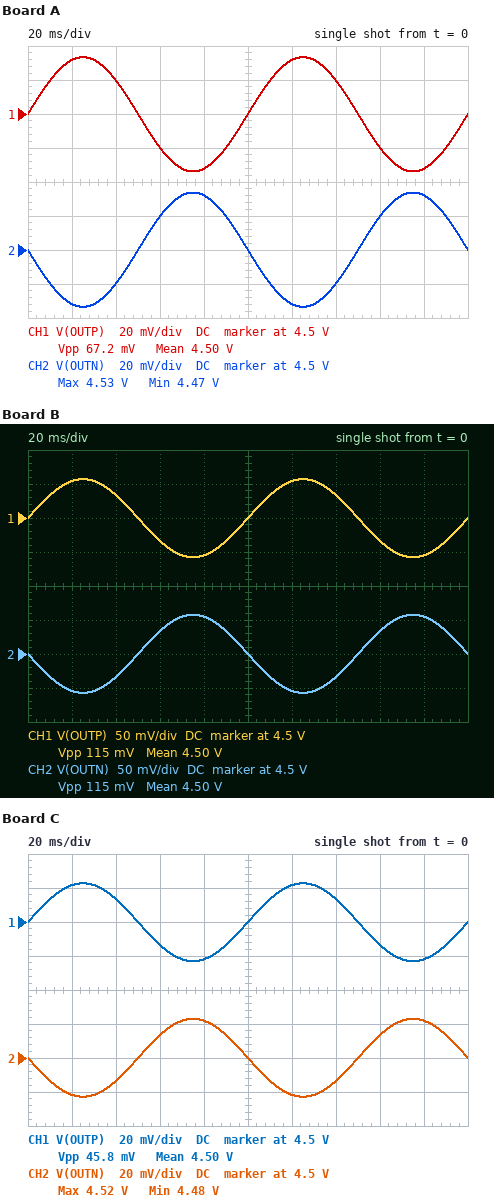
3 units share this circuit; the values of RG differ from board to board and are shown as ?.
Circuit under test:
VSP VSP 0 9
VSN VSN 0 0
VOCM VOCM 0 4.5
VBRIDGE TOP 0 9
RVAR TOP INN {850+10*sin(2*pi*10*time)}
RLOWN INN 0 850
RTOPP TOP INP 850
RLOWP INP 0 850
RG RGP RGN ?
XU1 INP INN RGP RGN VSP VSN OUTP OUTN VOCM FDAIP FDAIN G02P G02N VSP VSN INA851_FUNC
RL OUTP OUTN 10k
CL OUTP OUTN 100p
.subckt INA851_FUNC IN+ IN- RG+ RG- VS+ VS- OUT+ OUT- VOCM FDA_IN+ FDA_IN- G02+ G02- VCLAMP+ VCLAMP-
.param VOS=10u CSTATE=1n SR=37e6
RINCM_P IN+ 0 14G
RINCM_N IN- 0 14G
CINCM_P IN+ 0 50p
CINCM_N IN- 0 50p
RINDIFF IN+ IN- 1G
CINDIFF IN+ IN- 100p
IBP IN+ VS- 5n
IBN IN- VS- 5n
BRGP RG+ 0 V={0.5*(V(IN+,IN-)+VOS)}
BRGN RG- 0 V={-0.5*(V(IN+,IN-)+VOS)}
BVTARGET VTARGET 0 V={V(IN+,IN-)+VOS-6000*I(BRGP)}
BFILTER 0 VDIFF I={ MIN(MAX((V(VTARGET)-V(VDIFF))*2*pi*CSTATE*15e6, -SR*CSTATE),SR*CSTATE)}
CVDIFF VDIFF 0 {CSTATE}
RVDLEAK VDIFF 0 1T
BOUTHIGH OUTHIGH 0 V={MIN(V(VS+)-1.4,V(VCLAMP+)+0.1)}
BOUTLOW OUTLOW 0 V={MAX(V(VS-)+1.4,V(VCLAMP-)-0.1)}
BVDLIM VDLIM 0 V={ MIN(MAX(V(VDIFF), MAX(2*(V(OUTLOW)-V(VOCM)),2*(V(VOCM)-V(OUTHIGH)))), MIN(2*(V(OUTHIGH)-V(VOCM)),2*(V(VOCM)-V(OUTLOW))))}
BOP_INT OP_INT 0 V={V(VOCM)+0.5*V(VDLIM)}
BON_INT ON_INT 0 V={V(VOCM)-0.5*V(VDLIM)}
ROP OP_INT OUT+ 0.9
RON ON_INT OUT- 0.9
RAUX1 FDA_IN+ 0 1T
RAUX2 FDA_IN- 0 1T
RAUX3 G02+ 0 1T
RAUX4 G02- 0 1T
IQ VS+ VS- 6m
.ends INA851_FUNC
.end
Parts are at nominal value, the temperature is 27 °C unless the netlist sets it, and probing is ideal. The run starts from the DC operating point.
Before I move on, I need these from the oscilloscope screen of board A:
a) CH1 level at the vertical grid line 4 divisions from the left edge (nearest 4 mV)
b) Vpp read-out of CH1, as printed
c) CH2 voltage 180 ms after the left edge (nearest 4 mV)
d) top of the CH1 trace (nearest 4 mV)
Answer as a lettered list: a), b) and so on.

a) 4.468 V
b) 67.2 mV
c) 4.532 V
d) 4.532 V
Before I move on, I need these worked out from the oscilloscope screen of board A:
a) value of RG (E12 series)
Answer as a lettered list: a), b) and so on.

a) 3.9 kΩ
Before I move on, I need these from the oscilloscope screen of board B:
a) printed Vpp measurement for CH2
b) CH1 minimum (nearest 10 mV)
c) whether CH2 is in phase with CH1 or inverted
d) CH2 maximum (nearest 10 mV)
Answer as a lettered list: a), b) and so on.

a) 115 mV
b) 4.44 V
c) inverted
d) 4.56 V
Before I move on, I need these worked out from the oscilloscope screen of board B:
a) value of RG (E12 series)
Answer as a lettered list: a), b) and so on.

a) 1.8 kΩ
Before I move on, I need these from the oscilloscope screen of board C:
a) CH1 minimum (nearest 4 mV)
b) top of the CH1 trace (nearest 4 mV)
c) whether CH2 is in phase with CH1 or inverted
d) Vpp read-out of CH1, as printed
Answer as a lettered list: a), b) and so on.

a) 4.476 V
b) 4.524 V
c) inverted
d) 45.8 mV
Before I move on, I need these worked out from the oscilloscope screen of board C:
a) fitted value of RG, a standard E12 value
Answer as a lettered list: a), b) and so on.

a) 8.2 kΩ
